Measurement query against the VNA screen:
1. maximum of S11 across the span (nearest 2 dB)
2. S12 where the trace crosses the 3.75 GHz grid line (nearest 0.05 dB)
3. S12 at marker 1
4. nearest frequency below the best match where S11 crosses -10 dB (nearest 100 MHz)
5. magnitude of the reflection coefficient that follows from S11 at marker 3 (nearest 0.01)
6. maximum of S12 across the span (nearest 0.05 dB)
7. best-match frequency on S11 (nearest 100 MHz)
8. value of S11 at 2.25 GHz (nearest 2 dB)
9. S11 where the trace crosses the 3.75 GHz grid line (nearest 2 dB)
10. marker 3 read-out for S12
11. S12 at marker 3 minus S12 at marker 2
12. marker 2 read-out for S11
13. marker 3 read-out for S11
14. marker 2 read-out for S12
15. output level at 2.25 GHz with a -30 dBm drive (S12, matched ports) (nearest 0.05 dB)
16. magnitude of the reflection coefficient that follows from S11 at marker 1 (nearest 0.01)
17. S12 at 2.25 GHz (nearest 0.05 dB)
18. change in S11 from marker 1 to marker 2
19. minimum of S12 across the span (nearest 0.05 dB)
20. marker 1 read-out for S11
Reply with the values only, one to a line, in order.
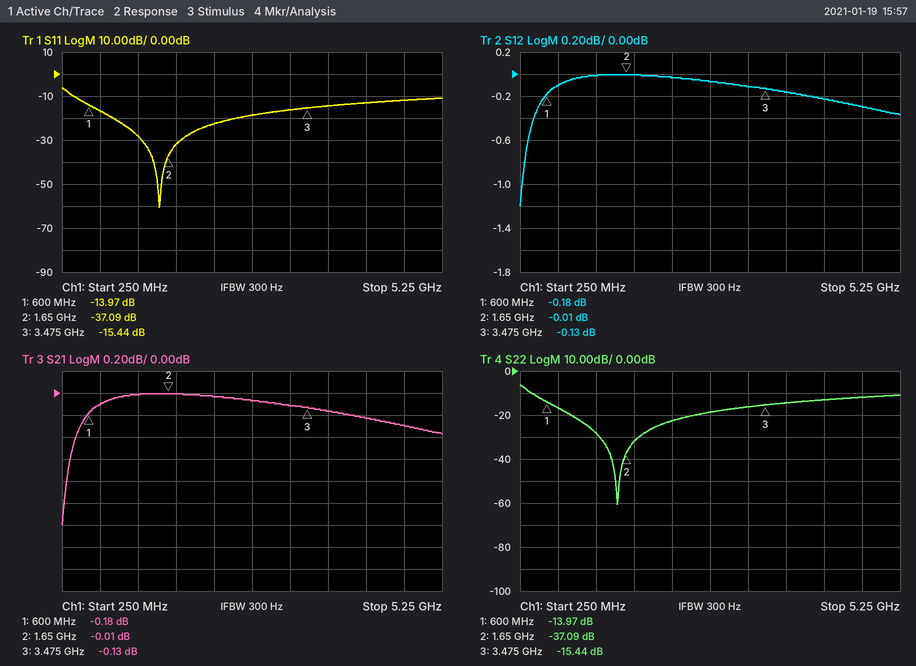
-6 dB
-0.15 dB
-0.18 dB
400 MHz
0.17
0.00 dB
1.5 GHz
-22 dB
-14 dB
-0.13 dB
-0.12 dB
-37.09 dB
-15.44 dB
-0.01 dB
-30.05 dBm
0.20
-0.05 dB
-23.12 dB
-1.20 dB
-13.97 dB
